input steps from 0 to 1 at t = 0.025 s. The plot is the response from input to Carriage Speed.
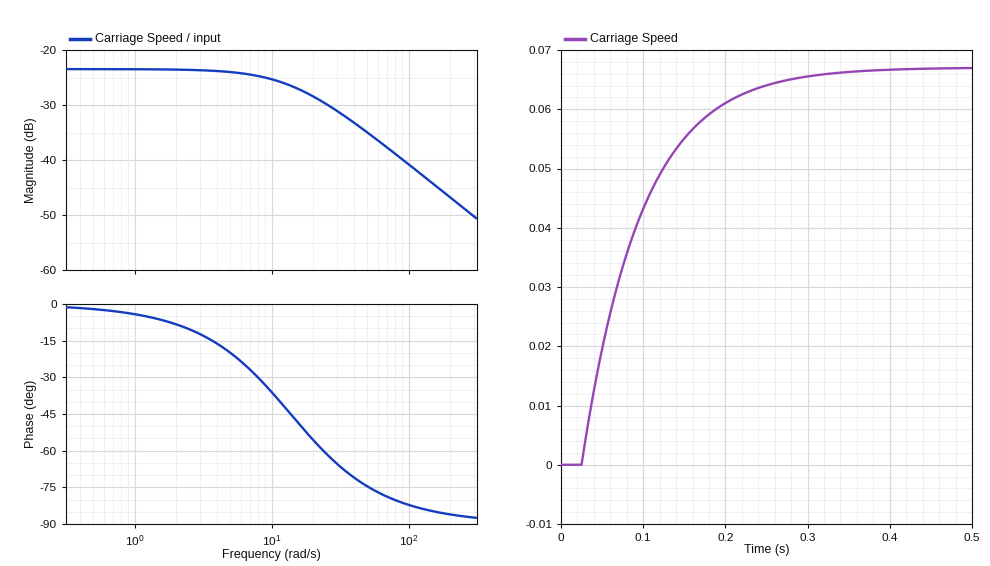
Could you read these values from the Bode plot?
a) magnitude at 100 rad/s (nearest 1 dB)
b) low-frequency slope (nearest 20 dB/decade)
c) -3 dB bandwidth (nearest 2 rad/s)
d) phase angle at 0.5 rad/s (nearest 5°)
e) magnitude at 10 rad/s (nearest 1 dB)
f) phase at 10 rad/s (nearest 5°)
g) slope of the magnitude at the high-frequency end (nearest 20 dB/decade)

-41 dB
0 dB/decade
14 rad/s
0°
-25 dB
-35°
-20 dB/decade
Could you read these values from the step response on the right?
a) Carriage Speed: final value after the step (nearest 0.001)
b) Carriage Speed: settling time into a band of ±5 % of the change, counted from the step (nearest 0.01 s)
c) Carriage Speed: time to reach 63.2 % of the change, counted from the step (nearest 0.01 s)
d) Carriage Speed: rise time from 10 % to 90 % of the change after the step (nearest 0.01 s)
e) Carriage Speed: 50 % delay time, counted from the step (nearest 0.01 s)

0.067
0.22 s
0.07 s
0.16 s
0.05 s
